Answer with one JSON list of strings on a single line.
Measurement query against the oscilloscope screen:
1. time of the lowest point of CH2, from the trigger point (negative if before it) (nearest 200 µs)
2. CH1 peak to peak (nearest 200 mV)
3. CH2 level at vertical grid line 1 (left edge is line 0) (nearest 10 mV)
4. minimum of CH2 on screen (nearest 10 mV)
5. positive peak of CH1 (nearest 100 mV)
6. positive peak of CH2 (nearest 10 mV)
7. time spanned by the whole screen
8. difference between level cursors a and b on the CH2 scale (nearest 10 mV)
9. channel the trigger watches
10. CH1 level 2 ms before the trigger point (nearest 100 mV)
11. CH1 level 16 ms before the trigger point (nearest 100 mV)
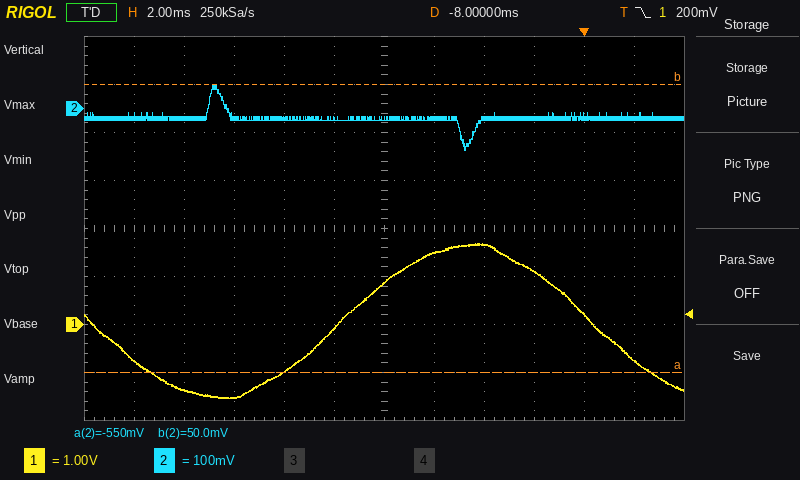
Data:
["-4.8 ms", "3.2 V", "-20 mV", "-90 mV", "1.7 V", "50 mV", "24 ms", "600 mV", "CH1", "1.1 V", "-1.4 V"]
